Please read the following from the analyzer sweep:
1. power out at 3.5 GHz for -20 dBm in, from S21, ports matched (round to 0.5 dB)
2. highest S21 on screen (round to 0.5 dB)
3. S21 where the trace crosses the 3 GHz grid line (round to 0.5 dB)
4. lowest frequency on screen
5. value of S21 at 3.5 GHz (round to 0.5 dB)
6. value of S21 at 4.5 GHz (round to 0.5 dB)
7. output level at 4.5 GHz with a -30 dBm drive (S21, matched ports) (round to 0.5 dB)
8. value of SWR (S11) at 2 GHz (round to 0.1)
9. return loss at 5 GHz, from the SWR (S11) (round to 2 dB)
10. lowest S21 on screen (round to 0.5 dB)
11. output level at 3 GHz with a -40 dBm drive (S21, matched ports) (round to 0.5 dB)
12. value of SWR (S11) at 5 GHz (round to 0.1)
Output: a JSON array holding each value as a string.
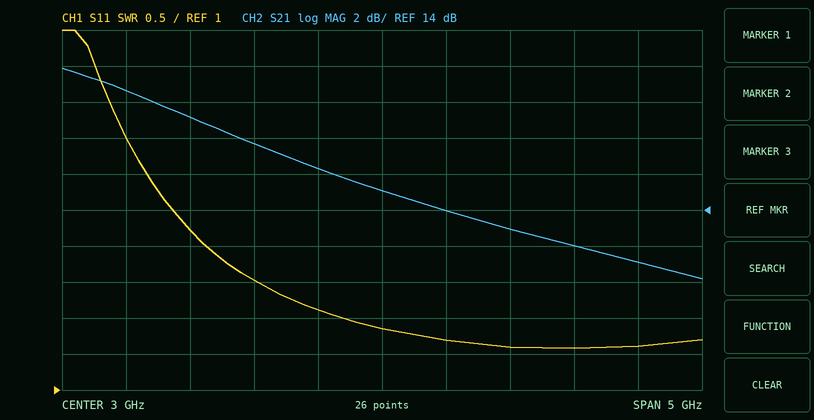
["-6.0 dBm", "22.0 dB", "15.0 dB", "500 MHz", "14.0 dB", "12.0 dB", "-18.0 dBm", "2.5", "12 dB", "10.0 dB", "-25.0 dBm", "1.6"]
